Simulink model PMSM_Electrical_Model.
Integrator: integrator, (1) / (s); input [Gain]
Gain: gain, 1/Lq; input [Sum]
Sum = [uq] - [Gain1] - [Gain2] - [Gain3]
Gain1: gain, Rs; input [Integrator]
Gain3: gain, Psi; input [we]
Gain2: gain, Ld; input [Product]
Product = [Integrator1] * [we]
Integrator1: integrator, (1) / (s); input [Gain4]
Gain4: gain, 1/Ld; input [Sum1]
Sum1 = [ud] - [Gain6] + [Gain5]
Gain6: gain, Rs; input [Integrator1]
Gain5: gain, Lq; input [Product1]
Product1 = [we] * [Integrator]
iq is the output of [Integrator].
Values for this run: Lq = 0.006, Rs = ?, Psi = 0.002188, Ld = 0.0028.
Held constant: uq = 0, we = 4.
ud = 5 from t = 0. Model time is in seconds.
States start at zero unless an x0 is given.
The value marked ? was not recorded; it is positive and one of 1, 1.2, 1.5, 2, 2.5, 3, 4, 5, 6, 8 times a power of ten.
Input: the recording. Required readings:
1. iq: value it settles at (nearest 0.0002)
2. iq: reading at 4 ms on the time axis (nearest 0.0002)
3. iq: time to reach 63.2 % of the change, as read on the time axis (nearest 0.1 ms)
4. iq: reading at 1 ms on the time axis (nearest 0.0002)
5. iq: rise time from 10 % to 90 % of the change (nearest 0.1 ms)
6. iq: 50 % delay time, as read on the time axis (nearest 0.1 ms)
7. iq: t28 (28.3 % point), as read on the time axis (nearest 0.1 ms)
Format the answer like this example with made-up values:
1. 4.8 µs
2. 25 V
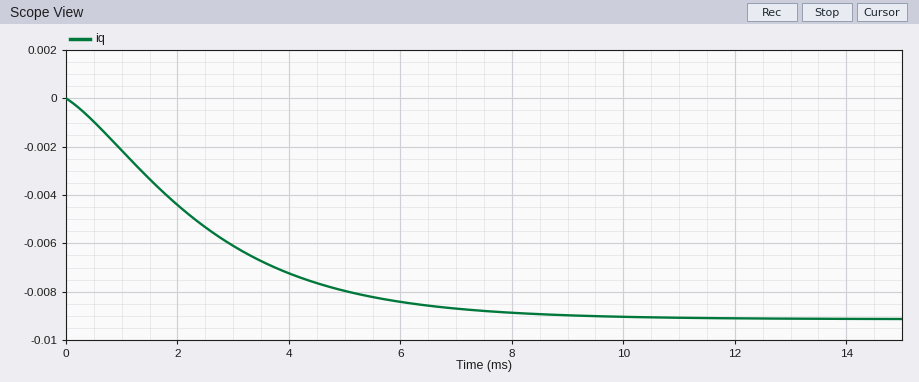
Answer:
1. -0.0092
2. -0.0072
3. 2.8 ms
4. -0.0022
5. 5.0 ms
6. 2.1 ms
7. 1.2 ms
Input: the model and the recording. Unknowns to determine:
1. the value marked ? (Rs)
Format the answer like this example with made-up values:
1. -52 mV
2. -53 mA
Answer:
1. 3
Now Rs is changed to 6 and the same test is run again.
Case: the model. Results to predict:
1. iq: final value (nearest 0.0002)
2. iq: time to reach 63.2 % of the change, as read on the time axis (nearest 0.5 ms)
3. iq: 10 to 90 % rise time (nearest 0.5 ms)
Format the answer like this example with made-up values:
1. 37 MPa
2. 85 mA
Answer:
1. -0.0030
2. 1.5 ms
3. 2.5 ms
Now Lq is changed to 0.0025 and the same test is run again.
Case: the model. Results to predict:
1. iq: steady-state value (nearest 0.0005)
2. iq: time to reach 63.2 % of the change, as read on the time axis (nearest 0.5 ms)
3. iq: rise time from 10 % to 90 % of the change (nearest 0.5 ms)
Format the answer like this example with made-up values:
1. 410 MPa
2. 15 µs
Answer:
1. -0.0090
2. 1.5 ms
3. 3.0 ms
